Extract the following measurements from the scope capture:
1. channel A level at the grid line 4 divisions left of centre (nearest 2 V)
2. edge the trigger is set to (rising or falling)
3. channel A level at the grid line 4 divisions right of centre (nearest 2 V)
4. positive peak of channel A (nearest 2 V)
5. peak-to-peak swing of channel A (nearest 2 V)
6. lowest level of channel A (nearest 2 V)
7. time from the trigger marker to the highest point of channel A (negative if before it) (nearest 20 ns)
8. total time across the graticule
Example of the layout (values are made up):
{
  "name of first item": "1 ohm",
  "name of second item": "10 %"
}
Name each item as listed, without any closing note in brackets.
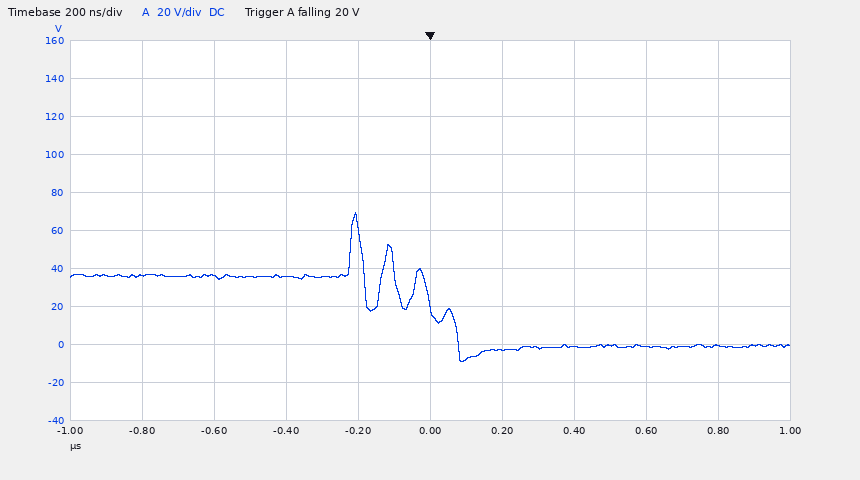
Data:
{
  "channel A level at the grid line 4 divisions left of centre": "36 V",
  "edge the trigger is set to": "falling",
  "channel A level at the grid line 4 divisions right of centre": "0 V",
  "positive peak of channel A": "70 V",
  "peak-to-peak swing of channel A": "78 V",
  "lowest level of channel A": "-8 V",
  "time from the trigger marker to the highest point of channel A (negative if before it)": "-200 ns",
  "total time across the graticule": "2 µs"
}
